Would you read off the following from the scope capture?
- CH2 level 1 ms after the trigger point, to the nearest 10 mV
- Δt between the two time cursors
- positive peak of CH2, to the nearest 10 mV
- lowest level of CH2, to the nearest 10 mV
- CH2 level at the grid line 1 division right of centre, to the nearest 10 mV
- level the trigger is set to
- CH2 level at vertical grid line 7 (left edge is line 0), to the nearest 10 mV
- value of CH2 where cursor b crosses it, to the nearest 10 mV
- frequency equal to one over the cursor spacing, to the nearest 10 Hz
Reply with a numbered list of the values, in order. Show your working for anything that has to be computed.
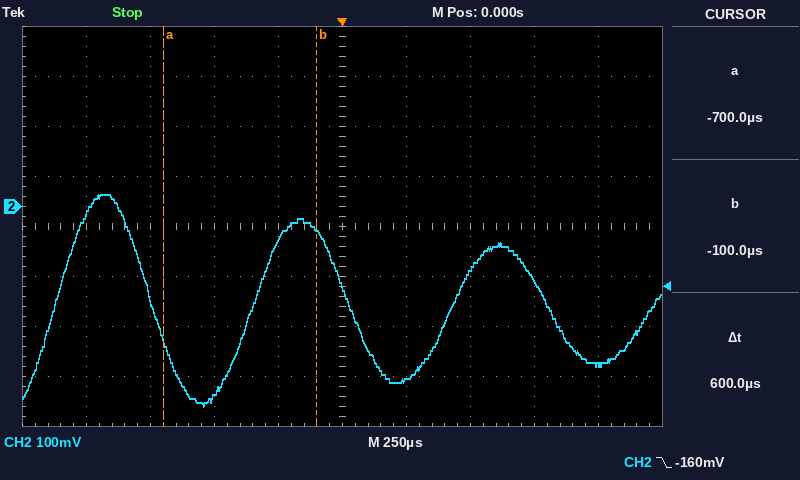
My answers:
1. -320 mV
2. 600 µs
3. 20 mV
4. -400 mV
5. -350 mV
6. -160 mV
7. -130 mV
8. -50 mV
9. 1 / 600 µs ≈ 1.67 kHz
